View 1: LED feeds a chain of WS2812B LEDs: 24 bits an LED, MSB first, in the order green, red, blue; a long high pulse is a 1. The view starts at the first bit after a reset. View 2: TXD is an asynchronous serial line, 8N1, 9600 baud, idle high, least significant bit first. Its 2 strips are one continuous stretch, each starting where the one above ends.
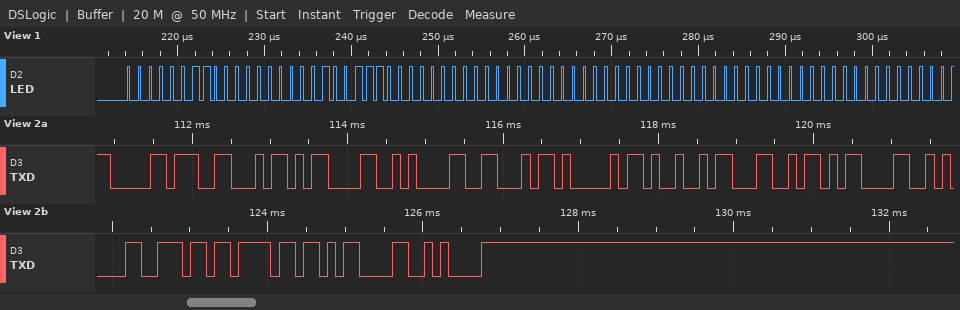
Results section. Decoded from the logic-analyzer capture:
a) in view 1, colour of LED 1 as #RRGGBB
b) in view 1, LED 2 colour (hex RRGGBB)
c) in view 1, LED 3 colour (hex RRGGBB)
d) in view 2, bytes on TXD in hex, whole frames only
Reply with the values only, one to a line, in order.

#000327
#000000
#000000
0xB0 0x46 0x0D 0x0A 0x46 0x41 0x49 0x4C 0x0D 0x0A 0x6E 0x6F 0x0D 0x0A
